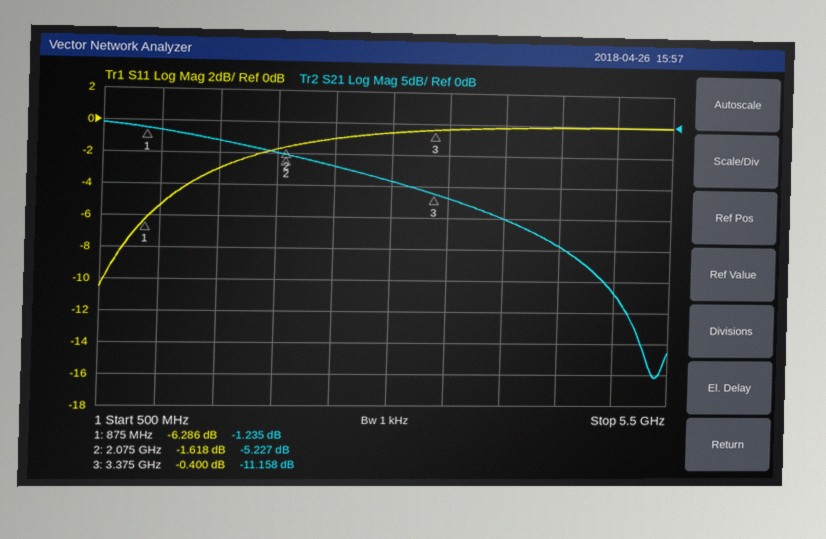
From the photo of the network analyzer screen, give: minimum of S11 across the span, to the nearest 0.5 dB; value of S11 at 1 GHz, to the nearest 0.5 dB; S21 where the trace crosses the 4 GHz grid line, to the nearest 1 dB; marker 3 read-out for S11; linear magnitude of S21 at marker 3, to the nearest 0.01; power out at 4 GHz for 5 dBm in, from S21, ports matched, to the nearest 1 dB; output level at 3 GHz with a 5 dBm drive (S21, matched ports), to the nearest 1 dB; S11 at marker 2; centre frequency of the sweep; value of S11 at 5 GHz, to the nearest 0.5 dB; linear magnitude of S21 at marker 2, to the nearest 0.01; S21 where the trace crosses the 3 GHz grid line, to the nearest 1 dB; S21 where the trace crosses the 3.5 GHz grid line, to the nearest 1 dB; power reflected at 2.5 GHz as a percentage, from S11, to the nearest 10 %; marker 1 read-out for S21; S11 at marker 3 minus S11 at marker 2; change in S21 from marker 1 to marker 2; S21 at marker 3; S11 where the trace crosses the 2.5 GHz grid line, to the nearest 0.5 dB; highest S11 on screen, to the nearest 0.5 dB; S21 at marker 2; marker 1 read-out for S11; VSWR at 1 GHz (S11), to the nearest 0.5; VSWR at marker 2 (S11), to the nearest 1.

-10.5 dB
-5.5 dB
-15 dB
-0.400 dB
0.28
-10 dBm
-4 dBm
-1.618 dB
3 GHz
0.0 dB
0.55
-9 dB
-12 dB
80 %
-1.235 dB
1.218 dB
-3.992 dB
-11.158 dB
-1.0 dB
0.0 dB
-5.227 dB
-6.286 dB
3.5
11
